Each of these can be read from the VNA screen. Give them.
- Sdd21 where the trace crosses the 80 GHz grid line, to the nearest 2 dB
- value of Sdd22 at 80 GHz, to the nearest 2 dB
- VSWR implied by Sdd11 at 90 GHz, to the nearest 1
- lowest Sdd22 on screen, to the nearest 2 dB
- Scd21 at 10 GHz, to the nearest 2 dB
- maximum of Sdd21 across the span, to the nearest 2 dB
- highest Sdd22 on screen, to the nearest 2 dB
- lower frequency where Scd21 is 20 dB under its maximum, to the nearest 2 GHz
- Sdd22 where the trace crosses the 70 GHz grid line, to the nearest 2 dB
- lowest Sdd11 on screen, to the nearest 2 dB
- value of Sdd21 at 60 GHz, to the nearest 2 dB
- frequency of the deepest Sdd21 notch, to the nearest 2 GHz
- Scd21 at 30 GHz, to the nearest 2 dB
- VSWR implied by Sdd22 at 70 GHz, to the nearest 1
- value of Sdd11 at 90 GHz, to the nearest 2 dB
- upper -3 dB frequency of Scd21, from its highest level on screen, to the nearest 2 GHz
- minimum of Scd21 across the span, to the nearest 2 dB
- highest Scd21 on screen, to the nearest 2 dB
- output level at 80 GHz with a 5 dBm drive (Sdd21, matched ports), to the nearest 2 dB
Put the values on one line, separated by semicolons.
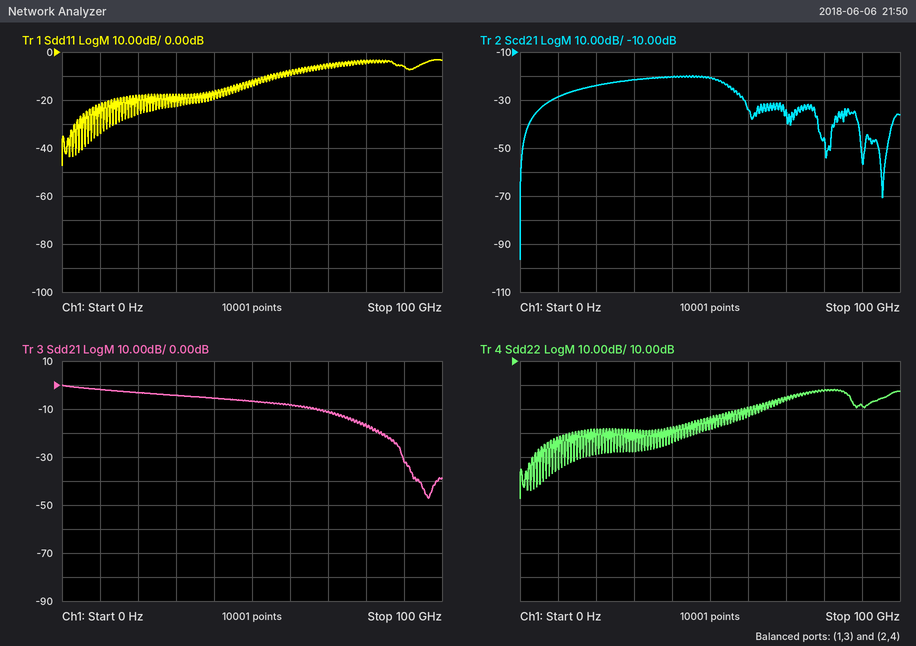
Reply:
-16 dB; -2 dB; 3; -48 dB; -28 dB; 0 dB; -2 dB; 2 GHz; -6 dB; -48 dB; -8 dB; 96 GHz; -22 dB; 3; -6 dB; 54 GHz; -96 dB; -20 dB; -12 dBm
